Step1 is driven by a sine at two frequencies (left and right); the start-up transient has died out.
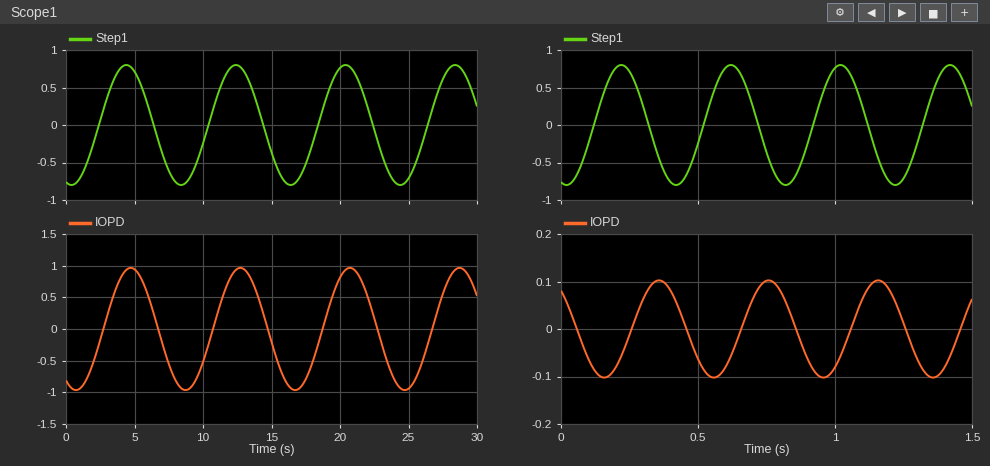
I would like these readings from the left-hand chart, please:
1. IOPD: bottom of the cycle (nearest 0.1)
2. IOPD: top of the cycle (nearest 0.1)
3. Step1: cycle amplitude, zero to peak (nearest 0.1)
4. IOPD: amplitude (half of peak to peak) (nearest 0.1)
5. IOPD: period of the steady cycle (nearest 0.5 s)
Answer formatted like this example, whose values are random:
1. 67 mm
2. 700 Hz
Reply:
1. -1.0
2. 1.0
3. 0.8
4. 1.0
5. 8.0 s
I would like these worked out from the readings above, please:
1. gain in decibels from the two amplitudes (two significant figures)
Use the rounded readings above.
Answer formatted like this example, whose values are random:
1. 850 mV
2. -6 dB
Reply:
1. 1.9 dB
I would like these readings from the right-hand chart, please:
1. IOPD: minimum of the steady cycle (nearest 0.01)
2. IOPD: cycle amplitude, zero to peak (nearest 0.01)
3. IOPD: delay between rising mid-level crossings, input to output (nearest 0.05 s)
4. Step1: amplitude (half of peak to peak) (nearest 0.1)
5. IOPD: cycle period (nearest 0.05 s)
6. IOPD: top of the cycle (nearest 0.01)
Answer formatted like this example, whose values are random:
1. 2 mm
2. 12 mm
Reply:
1. -0.10
2. 0.10
3. 0.15 s
4. 0.8
5. 0.40 s
6. 0.10
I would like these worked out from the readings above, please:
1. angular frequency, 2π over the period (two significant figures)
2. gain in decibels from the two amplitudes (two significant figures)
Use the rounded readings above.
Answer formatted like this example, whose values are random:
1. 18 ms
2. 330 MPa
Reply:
1. 16 rad/s
2. -18 dB
